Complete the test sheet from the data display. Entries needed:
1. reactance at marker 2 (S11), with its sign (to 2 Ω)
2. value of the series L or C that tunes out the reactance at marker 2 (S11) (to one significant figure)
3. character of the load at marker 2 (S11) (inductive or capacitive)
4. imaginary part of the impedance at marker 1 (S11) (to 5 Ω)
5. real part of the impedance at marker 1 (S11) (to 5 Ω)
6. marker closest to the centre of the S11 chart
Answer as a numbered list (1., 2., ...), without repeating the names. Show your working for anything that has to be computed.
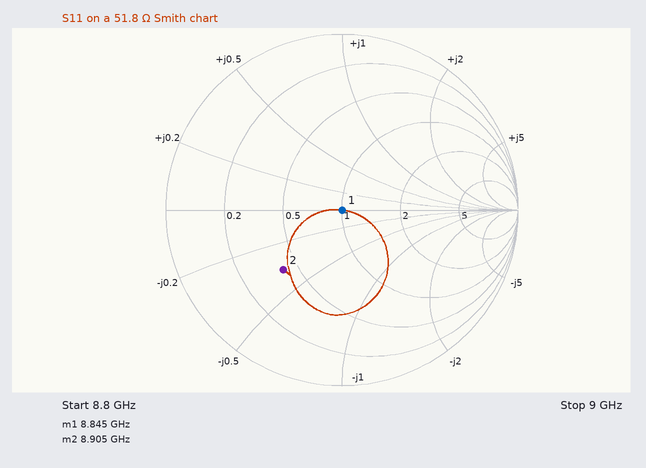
1. -18 Ω
2. L = 18 Ω/(2π × 8.905 GHz) ≈ 322 pH, so 300 pH to one significant figure
3. capacitive
4. 0 Ω
5. 50 Ω
6. marker 1
